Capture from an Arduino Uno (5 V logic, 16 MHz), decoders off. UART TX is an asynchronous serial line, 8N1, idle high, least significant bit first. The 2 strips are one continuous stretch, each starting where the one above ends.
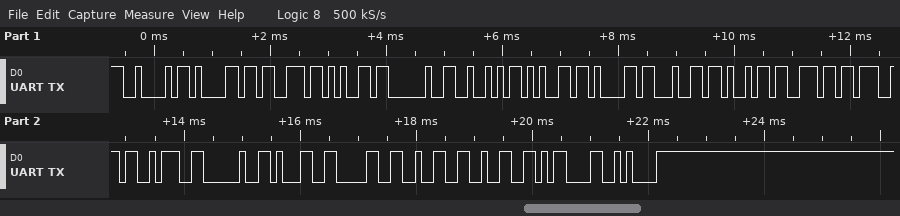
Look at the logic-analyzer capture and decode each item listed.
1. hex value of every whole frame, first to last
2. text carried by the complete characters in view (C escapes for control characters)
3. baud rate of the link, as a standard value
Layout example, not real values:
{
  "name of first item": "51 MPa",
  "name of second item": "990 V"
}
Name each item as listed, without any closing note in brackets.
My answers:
{
  "hex value of every whole frame, first to last": "42 61 73 65 20 52 65 61 64 69 6E 67 3A 20 31 30 32 32 0D 0A",
  "text carried by the complete characters in view": "\"Base Reading: 1022\\r\\n\"",
  "baud rate of the link, as a standard value": "9600 baud"
}
